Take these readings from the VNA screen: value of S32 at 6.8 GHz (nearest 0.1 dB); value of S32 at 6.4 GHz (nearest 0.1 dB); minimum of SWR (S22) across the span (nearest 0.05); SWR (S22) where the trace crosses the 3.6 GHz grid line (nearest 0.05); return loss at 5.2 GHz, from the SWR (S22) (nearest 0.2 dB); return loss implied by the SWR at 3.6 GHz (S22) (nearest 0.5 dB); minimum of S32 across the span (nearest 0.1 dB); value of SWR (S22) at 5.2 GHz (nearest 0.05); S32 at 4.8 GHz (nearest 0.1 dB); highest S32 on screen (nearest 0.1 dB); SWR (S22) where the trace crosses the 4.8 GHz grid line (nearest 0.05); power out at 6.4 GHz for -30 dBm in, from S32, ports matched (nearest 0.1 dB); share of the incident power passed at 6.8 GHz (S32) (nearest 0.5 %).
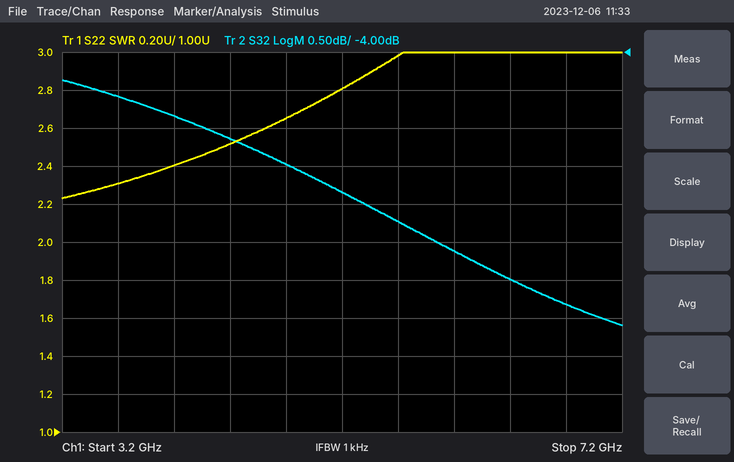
-7.3 dB
-7.0 dB
2.25
2.30
6.4 dB
8.0 dB
-7.6 dB
2.80
-5.5 dB
-4.4 dB
2.65
-37.0 dBm
18.5 %
